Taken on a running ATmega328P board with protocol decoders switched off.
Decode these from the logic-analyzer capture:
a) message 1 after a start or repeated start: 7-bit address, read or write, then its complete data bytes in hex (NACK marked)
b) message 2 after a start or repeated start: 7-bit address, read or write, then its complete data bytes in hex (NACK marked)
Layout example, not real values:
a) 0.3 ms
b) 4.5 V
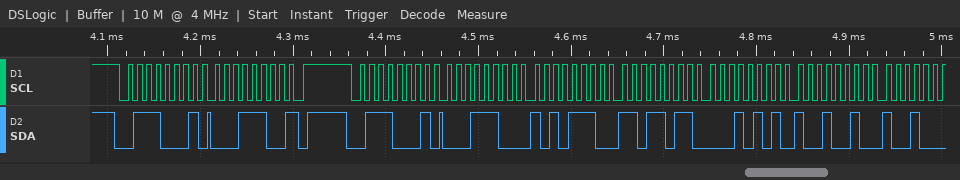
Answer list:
a) 0x38 read: 1C NACK
b) 0x38 read: 1C AE DB 15 92
